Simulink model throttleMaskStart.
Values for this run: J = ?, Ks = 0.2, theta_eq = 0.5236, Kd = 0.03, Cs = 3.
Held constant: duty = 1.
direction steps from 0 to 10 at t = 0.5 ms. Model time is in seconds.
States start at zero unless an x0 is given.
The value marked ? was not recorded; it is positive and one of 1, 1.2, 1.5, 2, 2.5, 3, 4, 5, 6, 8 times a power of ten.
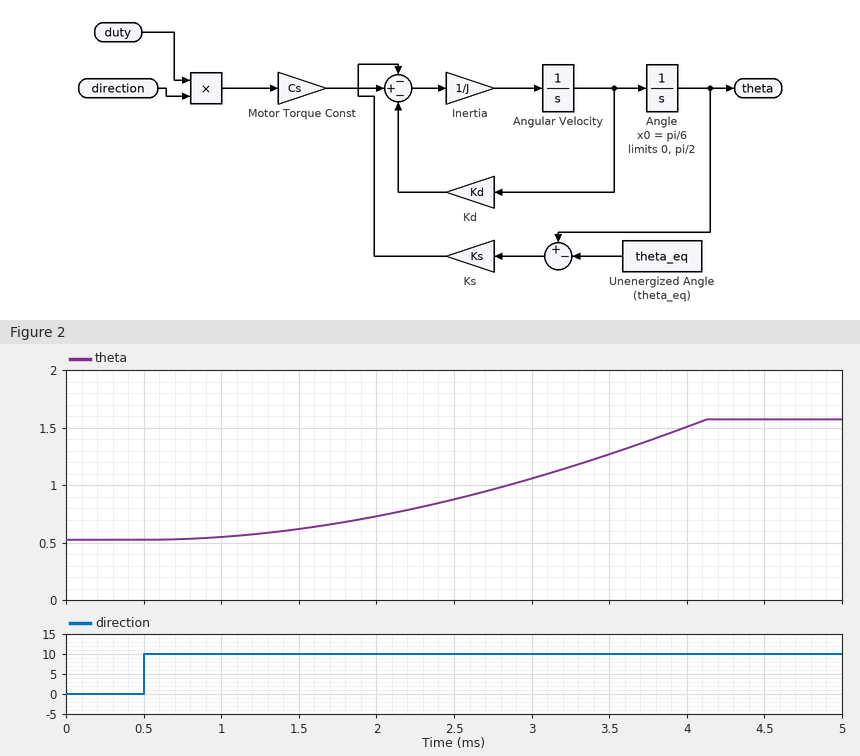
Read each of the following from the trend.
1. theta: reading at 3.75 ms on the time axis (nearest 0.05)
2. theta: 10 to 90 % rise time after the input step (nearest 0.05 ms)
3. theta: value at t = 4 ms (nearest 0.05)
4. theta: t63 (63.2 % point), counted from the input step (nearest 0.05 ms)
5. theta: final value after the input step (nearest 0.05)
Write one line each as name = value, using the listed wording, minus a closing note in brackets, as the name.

theta: reading at 3.75 ms on the time axis = 1.40
theta: 10 to 90 % rise time after the input step = 2.35 ms
theta: value at t = 4 ms = 1.50
theta: t63 (63.2 % point), counted from the input step = 2.80 ms
theta: final value after the input step = 1.55
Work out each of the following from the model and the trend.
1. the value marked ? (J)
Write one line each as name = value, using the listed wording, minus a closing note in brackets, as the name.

the value marked ? = 0.00015
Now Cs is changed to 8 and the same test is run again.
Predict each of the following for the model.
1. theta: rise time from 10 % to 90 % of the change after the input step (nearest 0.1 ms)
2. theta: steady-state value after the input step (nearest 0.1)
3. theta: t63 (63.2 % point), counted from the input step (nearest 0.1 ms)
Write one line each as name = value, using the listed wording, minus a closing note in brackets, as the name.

theta: rise time from 10 % to 90 % of the change after the input step = 1.4 ms
theta: steady-state value after the input step = 1.6
theta: t63 (63.2 % point), counted from the input step = 1.7 ms
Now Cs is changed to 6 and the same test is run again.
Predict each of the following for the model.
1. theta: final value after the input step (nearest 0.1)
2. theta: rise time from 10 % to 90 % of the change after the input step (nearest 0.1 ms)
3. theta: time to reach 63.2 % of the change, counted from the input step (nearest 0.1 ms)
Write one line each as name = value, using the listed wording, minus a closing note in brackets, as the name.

theta: final value after the input step = 1.6
theta: rise time from 10 % to 90 % of the change after the input step = 1.6 ms
theta: time to reach 63.2 % of the change, counted from the input step = 1.9 ms
